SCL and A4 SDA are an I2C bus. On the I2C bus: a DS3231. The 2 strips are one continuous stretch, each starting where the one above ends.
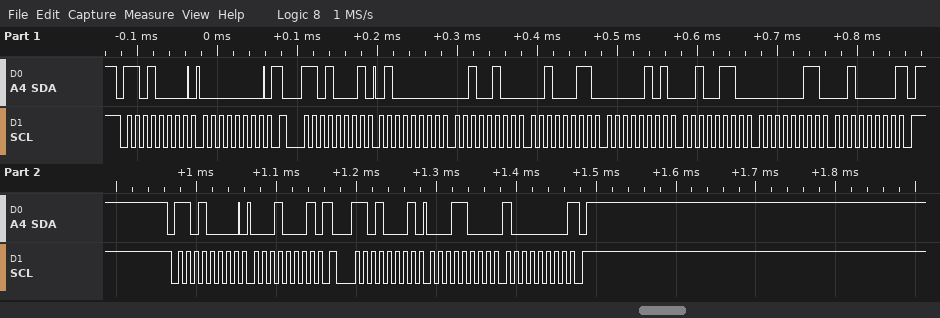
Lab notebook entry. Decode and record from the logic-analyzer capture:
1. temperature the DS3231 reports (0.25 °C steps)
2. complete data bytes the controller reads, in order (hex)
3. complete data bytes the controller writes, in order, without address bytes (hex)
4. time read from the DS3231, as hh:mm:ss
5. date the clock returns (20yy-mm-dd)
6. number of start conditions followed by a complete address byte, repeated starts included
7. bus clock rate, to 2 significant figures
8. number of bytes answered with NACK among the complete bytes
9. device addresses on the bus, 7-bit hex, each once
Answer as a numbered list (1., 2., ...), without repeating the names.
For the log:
1. 24.50 °C
2. 40 24 23 05 26 03 20 18 80
3. 00 11
4. 23:24:40
5. 2020-03-26
6. 4
7. 100 kHz
8. 2
9. 0x68
